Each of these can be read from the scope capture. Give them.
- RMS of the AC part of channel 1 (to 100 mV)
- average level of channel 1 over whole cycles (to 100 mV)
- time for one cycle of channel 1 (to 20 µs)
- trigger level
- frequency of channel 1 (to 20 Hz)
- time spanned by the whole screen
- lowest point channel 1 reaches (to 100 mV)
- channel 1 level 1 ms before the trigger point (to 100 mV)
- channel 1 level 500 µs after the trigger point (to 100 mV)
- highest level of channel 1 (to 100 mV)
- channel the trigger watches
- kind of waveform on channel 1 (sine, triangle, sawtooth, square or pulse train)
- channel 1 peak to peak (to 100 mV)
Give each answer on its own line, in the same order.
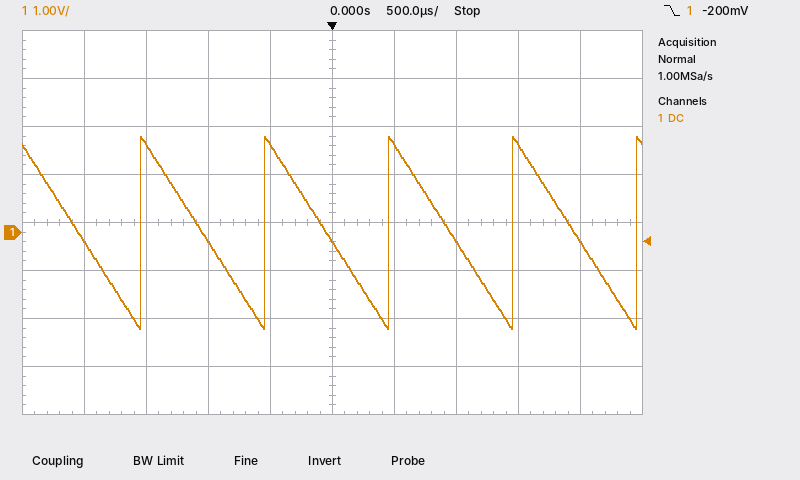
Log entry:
1.2 V
0.0 V
1.00 ms
-200 mV
1.00 kHz
5 ms
-2.0 V
-200 mV
1.8 V
2.0 V
channel 1
sawtooth
4.0 V
